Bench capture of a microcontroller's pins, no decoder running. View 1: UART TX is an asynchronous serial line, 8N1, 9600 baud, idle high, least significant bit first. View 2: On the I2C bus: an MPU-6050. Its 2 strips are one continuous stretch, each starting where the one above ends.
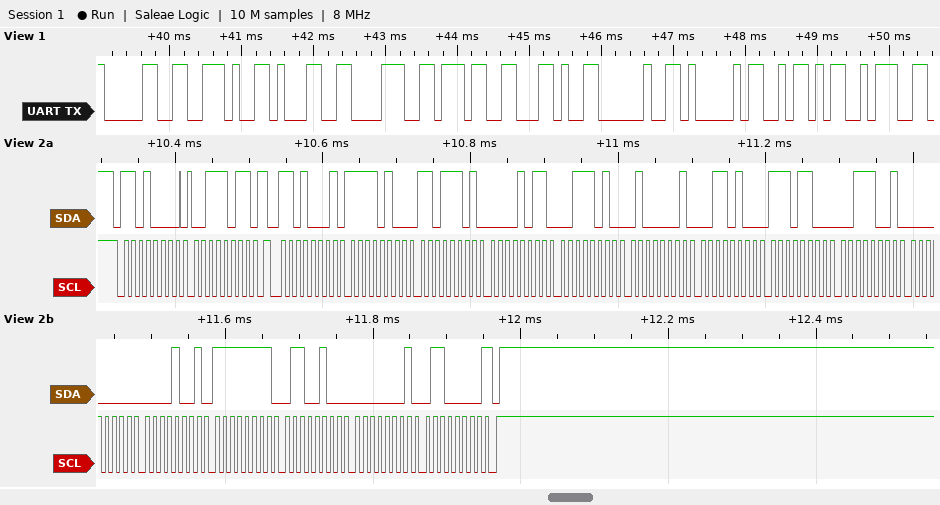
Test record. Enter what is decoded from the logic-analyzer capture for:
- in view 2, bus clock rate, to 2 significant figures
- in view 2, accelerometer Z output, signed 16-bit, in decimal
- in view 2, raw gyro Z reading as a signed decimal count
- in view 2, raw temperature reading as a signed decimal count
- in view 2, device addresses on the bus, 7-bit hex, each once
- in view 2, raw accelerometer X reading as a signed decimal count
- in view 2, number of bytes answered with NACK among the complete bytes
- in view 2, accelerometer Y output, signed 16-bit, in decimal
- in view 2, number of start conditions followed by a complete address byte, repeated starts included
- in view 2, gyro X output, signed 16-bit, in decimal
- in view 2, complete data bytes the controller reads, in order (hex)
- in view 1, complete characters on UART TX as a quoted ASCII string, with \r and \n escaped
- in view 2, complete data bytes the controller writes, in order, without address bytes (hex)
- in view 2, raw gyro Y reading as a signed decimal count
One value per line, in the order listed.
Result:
100 kHz
16692
352
-5063
0x68
-2851
1
2874
2
9
F4 DD 0B 3A 41 34 EC 39 00 09 FF 64 01 60
"0.187, AZ:"
3B
-156
